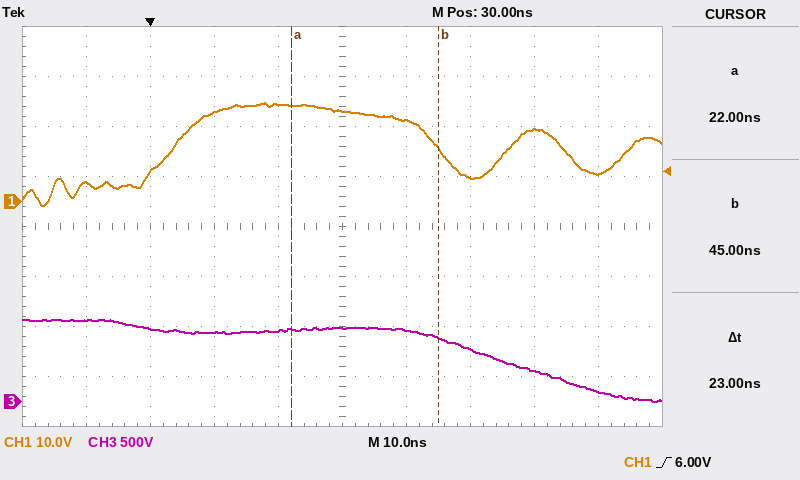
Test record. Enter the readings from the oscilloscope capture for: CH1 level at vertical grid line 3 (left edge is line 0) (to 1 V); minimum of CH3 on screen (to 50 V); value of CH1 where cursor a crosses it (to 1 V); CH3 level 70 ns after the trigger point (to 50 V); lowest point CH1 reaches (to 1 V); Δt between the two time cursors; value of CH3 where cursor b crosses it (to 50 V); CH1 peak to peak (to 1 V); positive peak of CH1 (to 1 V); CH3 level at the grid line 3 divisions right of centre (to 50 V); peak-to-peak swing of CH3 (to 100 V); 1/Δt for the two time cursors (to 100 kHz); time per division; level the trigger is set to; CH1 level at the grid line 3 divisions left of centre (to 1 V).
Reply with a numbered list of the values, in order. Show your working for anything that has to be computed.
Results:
1. 18 V
2. 0 V
3. 19 V
4. 100 V
5. -1 V
6. 23 ns
7. 650 V
8. 20 V − (-1 V) = 21 V
9. 20 V
10. 300 V
11. 800 V
12. 1 / 23 ns ≈ 43.5 MHz
13. 10 ns
14. 6.00 V
15. 6 V
